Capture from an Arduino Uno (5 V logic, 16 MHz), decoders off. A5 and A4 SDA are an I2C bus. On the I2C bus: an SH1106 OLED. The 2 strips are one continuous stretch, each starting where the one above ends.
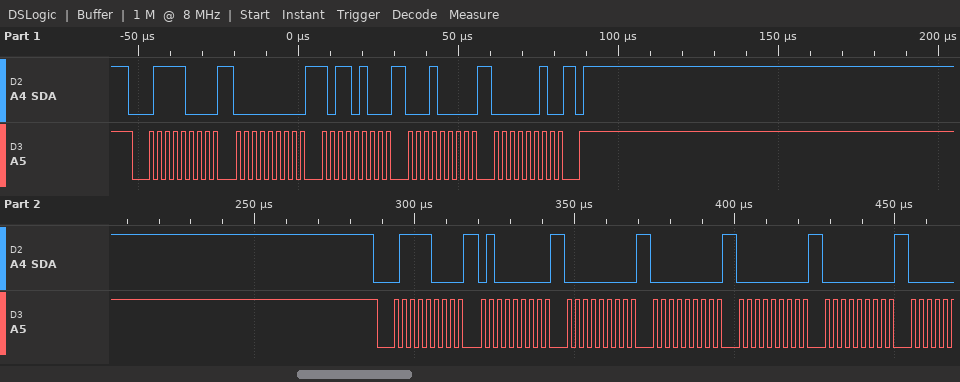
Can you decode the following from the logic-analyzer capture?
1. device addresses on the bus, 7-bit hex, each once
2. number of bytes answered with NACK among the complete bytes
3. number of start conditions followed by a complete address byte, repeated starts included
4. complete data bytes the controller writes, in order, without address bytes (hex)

0x3C
0
2
00 B4 10 02 40 00 00 00 00
